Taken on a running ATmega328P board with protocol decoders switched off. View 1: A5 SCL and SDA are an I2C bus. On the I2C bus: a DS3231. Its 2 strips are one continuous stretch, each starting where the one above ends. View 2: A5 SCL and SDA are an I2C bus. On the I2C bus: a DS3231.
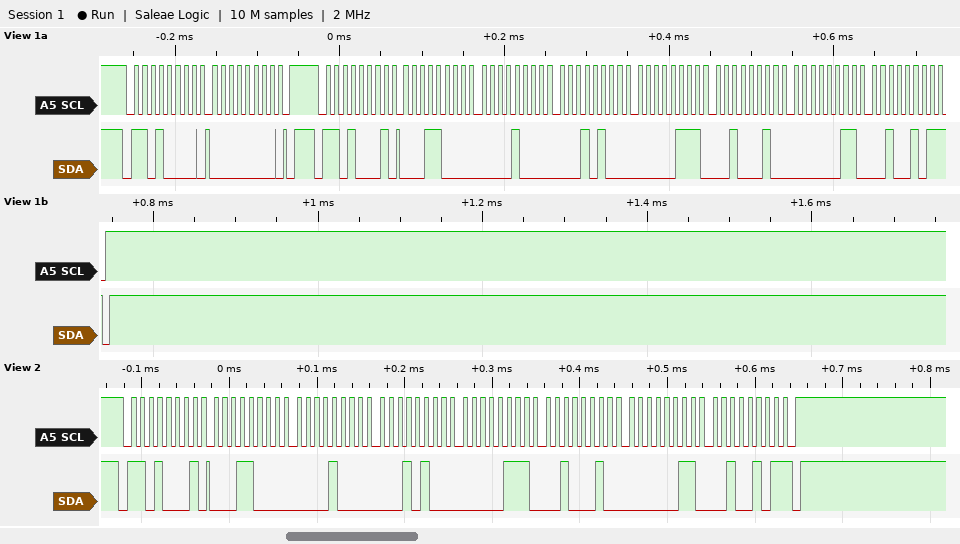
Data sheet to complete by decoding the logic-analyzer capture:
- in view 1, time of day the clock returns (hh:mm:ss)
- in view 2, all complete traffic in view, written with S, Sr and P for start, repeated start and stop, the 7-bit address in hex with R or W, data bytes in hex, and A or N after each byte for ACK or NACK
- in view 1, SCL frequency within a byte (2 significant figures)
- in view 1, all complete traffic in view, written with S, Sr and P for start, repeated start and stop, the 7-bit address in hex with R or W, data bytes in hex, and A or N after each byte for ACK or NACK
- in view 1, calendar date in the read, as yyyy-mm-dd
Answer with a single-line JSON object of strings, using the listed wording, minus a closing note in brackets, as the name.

{"in view 1, time of day the clock returns": "14:08:18", "in view 2, all complete traffic in view, written with S, Sr and P for start, repeated start and stop, the 7-bit address in hex with R or W, data bytes in hex, and A or N after each byte for ACK or NACK": "S 68R A 18 A 08 A 14 A 07 A 22 A 03 A 25 N P", "in view 1, SCL frequency within a byte": "100 kHz", "in view 1, all complete traffic in view, written with S, Sr and P for start, repeated start and stop, the 7-bit address in hex with R or W, data bytes in hex, and A or N after each byte for ACK or NACK": "S 68W A 00 A P S 68R A 18 A 08 A 14 A 07 A 22 A 03 A 25 N P", "in view 1, calendar date in the read, as yyyy-mm-dd": "2025-03-22"}
